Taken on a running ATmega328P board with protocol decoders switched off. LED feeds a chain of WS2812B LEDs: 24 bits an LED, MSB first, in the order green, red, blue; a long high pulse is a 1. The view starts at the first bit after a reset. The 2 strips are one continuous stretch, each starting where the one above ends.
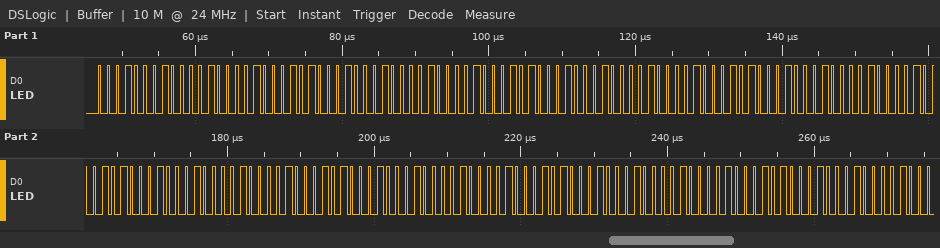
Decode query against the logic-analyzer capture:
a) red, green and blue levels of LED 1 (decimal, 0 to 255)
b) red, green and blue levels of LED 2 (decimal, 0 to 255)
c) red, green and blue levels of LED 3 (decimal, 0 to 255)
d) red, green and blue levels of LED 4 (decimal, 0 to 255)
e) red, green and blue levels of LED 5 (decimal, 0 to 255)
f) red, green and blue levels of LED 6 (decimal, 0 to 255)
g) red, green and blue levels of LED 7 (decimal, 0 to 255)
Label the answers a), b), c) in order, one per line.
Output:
a) 8, 17, 69
b) 8, 17, 69
c) 8, 17, 69
d) 8, 17, 69
e) 8, 17, 69
f) 8, 17, 69
g) 8, 17, 69
